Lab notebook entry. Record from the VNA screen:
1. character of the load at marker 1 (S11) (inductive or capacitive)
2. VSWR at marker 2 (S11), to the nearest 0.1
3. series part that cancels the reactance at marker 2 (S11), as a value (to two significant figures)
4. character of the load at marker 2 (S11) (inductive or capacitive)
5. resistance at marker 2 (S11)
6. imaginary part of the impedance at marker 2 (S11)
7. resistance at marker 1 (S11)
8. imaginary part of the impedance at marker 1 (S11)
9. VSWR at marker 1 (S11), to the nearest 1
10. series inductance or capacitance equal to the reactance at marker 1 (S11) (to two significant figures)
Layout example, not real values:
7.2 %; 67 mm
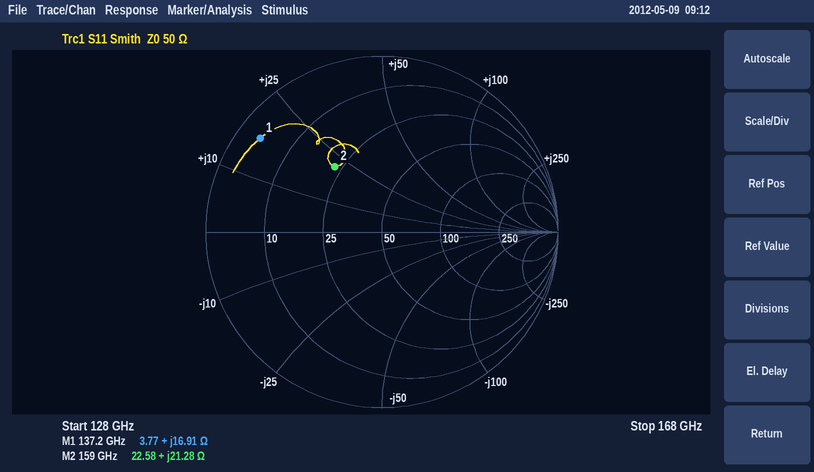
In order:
inductive; 2.7; 47 fF; inductive; 22.58 Ω; +21.28 Ω; 3.77 Ω; +16.91 Ω; 15; 20 pH
